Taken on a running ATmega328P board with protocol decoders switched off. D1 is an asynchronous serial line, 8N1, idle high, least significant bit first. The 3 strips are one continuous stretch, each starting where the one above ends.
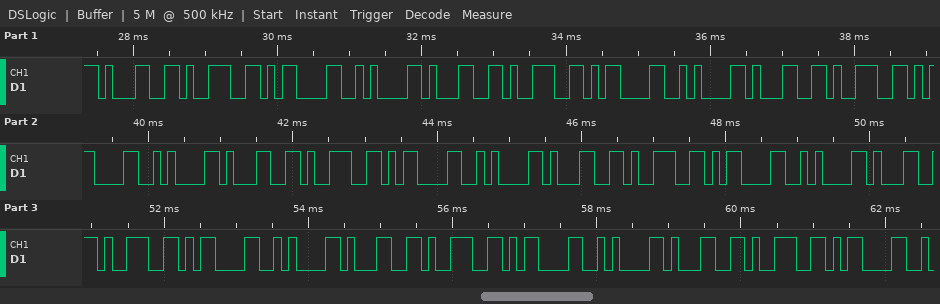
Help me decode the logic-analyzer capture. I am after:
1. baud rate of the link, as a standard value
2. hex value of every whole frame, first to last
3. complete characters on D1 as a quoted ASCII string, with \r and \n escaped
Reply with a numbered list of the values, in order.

1. 9600 baud
2. 31 39 0D 0A 31 39 0D 0A 31 39 0D 0A 31 39 0D 0A 31 39 0D 0A 31 39 0D 0A 31 39 0D 0A 31 39 0D
3. "19\r\n19\r\n19\r\n19\r\n19\r\n19\r\n19\r\n19\r"
